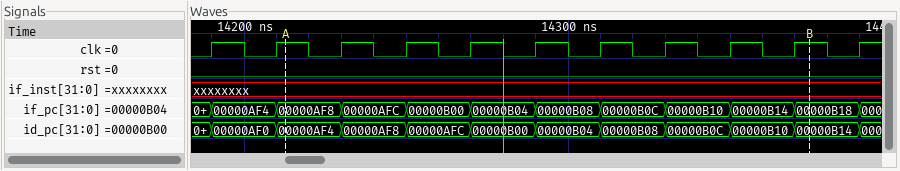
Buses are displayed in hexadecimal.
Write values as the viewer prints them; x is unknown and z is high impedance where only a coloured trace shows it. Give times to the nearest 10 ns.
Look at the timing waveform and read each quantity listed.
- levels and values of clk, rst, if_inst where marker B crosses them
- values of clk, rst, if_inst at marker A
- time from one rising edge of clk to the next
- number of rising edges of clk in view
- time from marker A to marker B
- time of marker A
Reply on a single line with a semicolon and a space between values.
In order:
clk=1, rst=0, if_inst=xxxxxxxx; clk=1, rst=0, if_inst=xxxxxxxx; 20 ns; 11; 160 ns; 14210 ns
